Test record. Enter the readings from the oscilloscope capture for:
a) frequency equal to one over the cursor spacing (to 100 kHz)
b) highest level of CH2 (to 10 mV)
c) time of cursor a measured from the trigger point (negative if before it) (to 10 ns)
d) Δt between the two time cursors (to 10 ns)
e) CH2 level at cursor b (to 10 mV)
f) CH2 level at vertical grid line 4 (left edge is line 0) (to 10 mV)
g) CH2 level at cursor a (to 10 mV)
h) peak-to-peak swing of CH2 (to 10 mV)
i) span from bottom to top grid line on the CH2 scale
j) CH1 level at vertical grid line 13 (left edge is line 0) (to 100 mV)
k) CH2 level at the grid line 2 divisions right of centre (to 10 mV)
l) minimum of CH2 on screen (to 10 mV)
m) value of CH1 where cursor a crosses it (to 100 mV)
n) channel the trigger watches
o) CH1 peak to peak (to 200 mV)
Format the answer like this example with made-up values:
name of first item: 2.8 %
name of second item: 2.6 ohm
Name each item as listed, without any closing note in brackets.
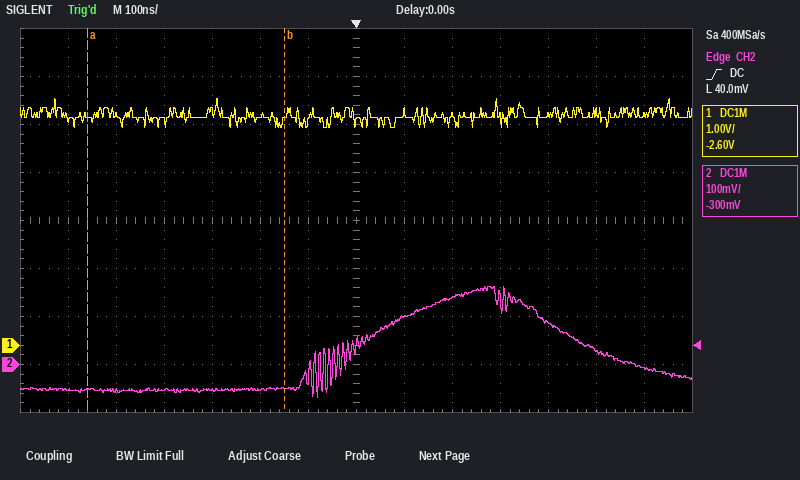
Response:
frequency equal to one over the cursor spacing: 2.4 MHz
highest level of CH2: 160 mV
time of cursor a measured from the trigger point (negative if before it): -560 ns
Δt between the two time cursors: 410 ns
CH2 level at cursor b: -50 mV
CH2 level at vertical grid line 4 (left edge is line 0): -50 mV
CH2 level at cursor a: -50 mV
peak-to-peak swing of CH2: 230 mV
span from bottom to top grid line on the CH2 scale: 800 mV
CH1 level at vertical grid line 13 (left edge is line 0): 4.8 V
CH2 level at the grid line 2 divisions right of centre: 140 mV
minimum of CH2 on screen: -70 mV
value of CH1 where cursor a crosses it: 4.8 V
channel the trigger watches: CH2
CH1 peak to peak: 600 mV
